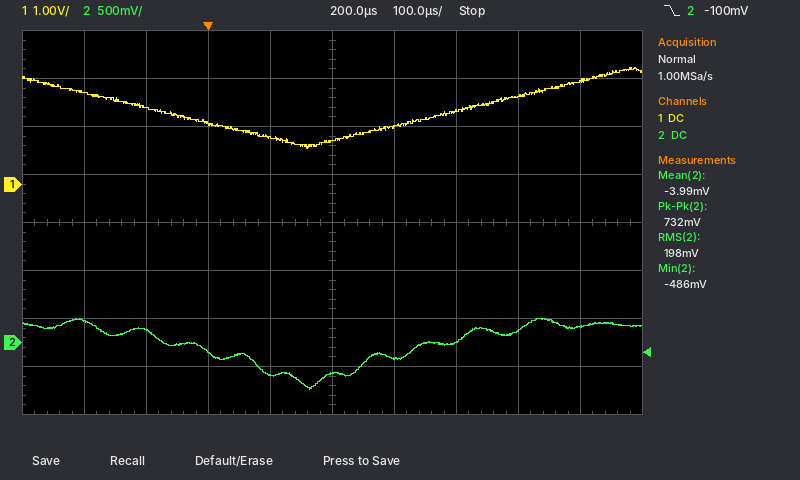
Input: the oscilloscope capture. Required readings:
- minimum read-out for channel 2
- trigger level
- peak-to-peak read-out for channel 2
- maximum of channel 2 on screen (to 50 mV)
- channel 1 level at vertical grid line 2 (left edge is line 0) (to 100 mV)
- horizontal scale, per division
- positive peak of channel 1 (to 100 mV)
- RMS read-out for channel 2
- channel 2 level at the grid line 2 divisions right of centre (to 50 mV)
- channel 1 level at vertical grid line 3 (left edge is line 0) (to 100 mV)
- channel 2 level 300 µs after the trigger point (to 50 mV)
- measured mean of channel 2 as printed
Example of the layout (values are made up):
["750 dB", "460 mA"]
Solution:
["-486 mV", "-100 mV", "732 mV", "250 mV", "1.6 V", "100 µs", "2.4 V", "198 mV", "0 mV", "1.3 V", "-150 mV", "-3.99 mV"]
